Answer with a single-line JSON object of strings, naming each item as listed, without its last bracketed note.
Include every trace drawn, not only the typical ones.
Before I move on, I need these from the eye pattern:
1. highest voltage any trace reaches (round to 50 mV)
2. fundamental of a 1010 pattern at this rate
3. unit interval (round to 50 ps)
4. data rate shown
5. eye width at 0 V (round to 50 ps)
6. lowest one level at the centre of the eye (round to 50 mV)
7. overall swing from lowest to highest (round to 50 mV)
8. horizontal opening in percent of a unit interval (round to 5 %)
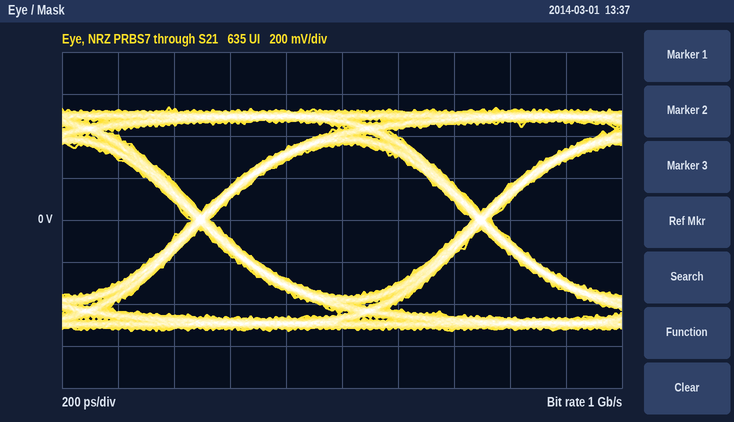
{"highest voltage any trace reaches": "550 mV", "fundamental of a 1010 pattern at this rate": "500 MHz", "unit interval": "1.00 ns", "data rate shown": "1 Gb/s", "eye width at 0 V": "950 ps", "lowest one level at the centre of the eye": "350 mV", "overall swing from lowest to highest": "1.05 V", "horizontal opening in percent of a unit interval": "95 %"}
